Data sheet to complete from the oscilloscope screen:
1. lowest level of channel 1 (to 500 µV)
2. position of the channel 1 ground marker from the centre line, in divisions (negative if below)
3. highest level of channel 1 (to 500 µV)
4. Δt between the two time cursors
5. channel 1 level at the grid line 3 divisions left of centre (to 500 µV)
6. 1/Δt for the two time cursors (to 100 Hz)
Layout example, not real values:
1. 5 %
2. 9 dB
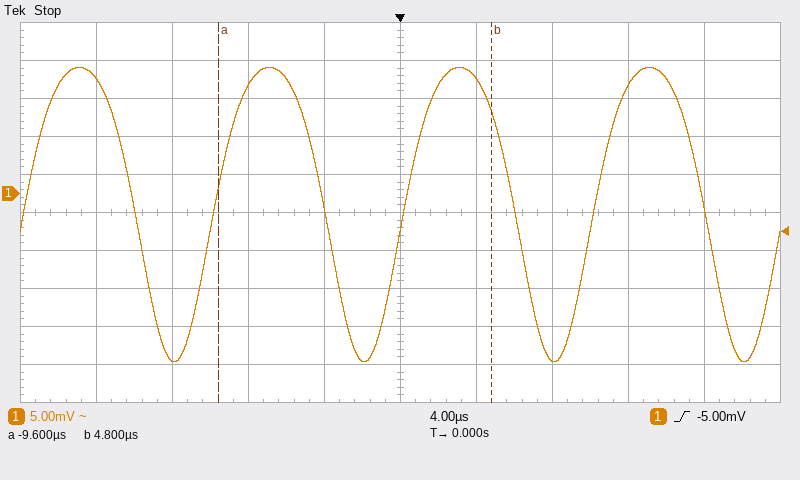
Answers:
1. -22.0 mV
2. +0.5 div
3. 16.5 mV
4. 14.4 µs
5. -22.0 mV
6. 69.4 kHz
